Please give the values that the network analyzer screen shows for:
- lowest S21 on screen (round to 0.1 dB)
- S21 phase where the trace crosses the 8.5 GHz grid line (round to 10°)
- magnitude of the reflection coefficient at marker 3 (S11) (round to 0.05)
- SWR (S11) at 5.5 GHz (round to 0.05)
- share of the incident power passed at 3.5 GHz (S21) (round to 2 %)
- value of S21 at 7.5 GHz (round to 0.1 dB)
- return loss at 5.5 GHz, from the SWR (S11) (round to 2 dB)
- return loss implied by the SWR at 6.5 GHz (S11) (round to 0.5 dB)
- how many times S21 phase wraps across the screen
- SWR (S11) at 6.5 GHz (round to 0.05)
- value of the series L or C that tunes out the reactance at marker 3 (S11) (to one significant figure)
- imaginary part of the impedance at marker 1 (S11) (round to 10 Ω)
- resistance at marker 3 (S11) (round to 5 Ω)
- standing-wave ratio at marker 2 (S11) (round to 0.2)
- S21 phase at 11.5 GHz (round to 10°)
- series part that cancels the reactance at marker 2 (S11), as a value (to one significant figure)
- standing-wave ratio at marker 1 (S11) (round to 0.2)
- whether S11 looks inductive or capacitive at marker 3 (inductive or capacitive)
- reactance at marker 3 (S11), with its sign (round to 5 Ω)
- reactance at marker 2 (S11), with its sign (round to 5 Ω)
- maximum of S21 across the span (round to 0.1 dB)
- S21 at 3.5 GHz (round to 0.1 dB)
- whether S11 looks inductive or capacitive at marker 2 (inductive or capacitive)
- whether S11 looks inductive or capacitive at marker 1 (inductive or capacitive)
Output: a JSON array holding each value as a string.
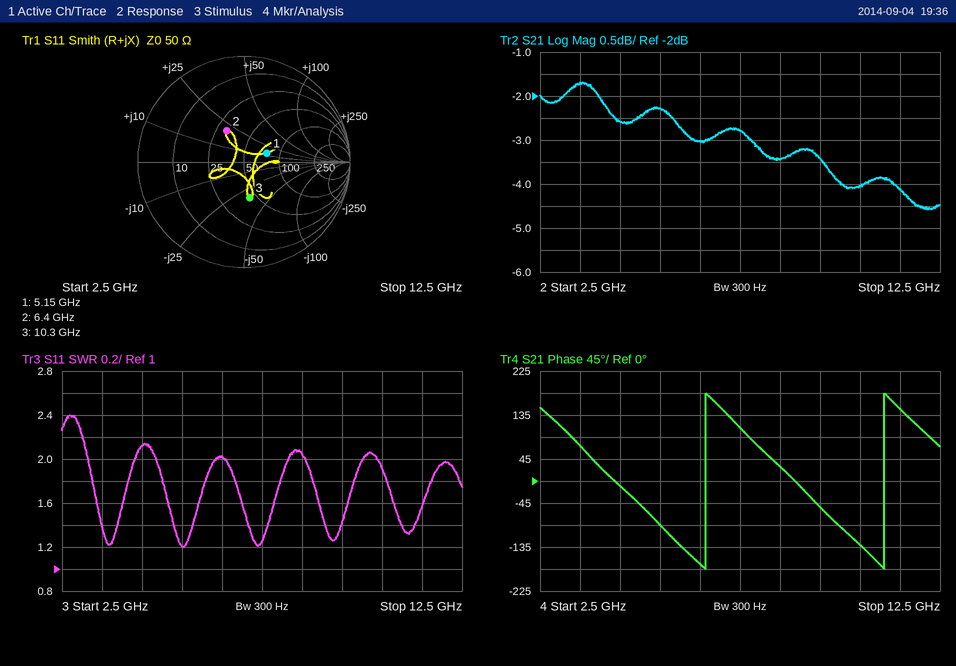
["-4.6 dB", "30°", "0.35", "1.20", "68 %", "-2.8 dB", "20 dB", "9.5 dB", "2", "2.00", "500 pH", "+10 Ω", "45 Ω", "2.0", "150°", "1 pF", "1.6", "capacitive", "-35 Ω", "+20 Ω", "-1.7 dB", "-1.7 dB", "inductive", "inductive"]
